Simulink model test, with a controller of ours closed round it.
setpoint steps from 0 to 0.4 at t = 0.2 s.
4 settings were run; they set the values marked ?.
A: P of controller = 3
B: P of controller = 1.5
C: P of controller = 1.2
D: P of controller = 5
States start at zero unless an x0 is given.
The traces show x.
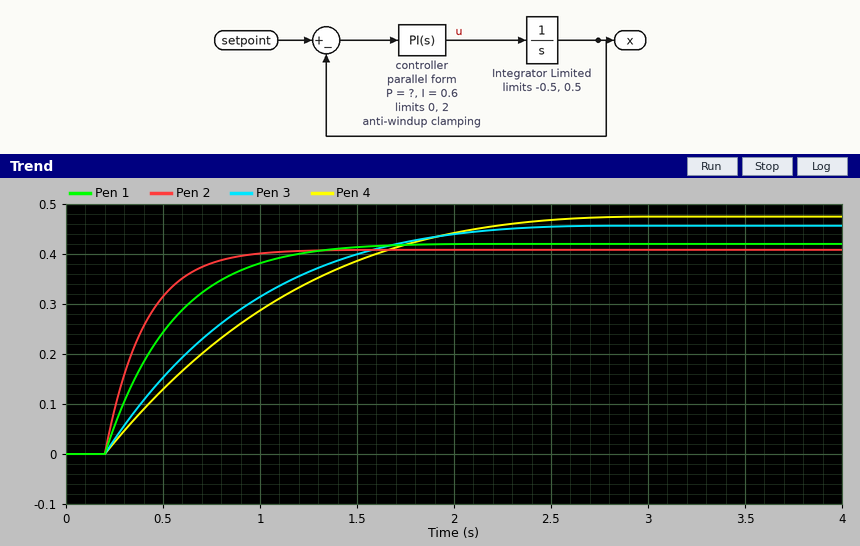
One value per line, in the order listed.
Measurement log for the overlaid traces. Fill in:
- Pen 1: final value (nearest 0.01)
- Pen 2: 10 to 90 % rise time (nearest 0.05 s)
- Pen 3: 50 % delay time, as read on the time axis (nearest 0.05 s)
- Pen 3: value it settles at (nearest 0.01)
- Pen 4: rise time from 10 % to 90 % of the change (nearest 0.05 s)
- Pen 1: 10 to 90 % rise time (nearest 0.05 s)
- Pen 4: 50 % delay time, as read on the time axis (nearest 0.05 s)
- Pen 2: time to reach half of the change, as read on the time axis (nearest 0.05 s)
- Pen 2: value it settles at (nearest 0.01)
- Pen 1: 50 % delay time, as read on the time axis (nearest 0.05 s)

0.42
0.45 s
0.70 s
0.46
1.55 s
0.75 s
0.80 s
0.35 s
0.41
0.45 s
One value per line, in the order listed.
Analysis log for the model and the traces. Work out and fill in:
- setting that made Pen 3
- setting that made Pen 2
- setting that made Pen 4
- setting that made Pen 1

B
D
C
A
